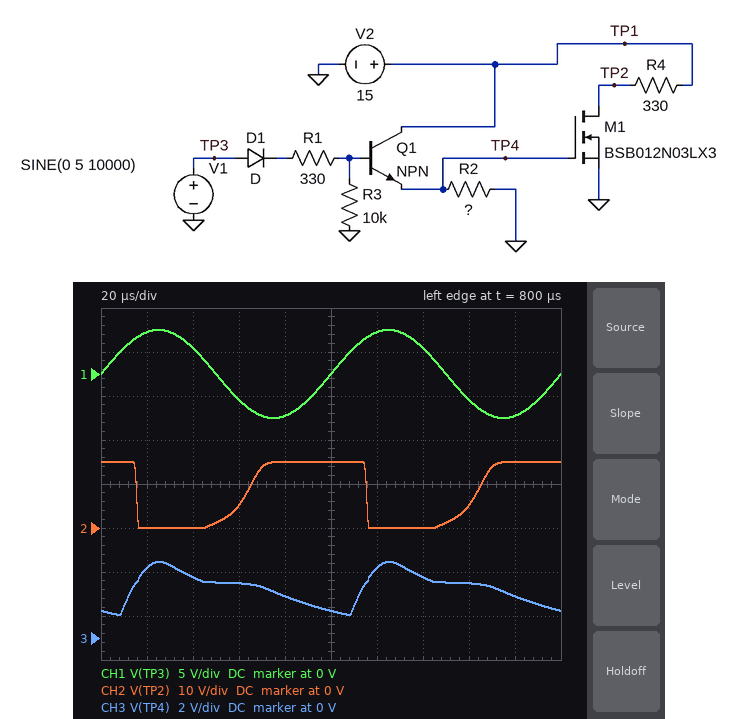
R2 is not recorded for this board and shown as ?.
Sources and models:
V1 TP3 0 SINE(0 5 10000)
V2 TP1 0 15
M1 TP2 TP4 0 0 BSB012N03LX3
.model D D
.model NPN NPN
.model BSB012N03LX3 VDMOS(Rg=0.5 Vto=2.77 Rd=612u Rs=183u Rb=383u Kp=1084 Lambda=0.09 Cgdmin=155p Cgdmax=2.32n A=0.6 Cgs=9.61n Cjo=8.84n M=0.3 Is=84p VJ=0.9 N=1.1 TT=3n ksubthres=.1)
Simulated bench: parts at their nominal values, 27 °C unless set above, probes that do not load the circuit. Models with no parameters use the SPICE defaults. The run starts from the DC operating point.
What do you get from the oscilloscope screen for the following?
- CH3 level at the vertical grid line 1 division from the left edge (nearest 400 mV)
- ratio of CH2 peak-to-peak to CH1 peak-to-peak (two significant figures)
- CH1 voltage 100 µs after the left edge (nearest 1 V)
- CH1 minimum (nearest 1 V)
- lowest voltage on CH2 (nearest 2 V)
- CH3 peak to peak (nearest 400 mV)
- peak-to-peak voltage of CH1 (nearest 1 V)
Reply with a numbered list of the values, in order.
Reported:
1. 3.2 V
2. 1.5
3. 0 V
4. -5 V
5. 0 V
6. 2.4 V
7. 10 V
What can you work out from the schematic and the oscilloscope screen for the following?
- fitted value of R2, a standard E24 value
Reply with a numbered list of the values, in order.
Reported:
1. 4.7 kΩ
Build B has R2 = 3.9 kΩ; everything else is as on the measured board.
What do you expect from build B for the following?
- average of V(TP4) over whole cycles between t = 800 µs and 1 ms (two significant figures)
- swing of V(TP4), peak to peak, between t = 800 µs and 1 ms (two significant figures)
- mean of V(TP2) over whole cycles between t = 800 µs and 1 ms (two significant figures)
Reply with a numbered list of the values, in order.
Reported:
1. 2.1 V
2. 2.7 V
3. 8.9 V
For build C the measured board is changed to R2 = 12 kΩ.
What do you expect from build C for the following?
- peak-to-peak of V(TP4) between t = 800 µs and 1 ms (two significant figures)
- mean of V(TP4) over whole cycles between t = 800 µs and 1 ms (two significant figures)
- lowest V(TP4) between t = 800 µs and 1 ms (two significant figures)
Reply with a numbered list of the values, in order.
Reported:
1. 1.0 V
2. 2.8 V
3. 2.5 V
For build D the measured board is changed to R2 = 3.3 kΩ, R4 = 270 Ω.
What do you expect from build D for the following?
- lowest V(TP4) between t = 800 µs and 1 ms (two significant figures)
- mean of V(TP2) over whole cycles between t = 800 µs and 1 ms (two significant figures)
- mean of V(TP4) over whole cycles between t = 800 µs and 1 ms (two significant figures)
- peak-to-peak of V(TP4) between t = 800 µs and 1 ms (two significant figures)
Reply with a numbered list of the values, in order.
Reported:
1. 530 mV
2. 9.6 V
3. 1.9 V
4. 2.9 V
